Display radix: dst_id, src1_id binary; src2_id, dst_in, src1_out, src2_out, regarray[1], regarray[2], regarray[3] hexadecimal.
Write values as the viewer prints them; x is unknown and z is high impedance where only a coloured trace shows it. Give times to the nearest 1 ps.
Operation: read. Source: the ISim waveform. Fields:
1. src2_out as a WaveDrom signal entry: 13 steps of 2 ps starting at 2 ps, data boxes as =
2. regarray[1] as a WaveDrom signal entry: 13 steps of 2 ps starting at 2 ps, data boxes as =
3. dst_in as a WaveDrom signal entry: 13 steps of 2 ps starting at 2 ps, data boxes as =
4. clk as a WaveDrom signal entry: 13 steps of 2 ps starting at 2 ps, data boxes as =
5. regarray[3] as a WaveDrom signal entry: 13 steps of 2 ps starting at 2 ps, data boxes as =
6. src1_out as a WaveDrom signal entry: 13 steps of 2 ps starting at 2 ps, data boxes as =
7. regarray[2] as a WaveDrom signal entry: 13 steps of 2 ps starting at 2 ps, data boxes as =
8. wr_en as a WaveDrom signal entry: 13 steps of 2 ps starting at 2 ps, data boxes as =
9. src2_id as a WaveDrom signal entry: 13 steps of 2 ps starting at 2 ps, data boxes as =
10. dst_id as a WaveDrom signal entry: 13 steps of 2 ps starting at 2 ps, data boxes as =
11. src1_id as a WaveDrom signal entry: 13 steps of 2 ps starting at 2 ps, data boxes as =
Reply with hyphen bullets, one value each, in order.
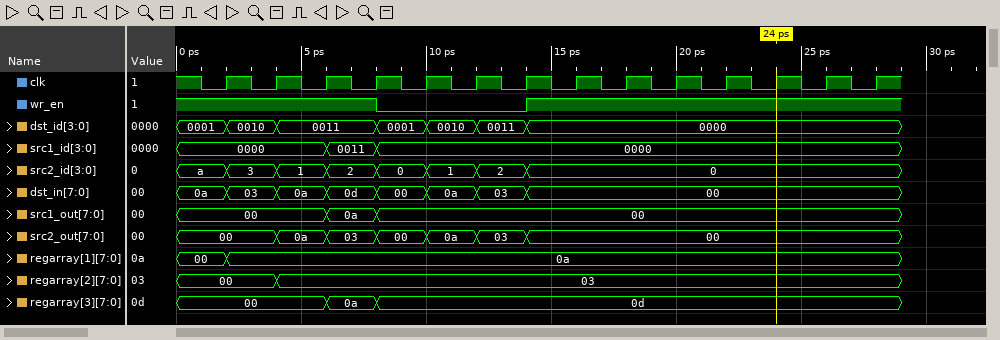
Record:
- {name: 'src2_out', wave: '=======......', data: '00 0a 03 00 0a 03 00'}
- {name: 'regarray[1]', wave: '=............', data: '0a'}
- {name: 'dst_in', wave: '=======......', data: '03 0a 0d 00 0a 03 00'}
- {name: 'clk', wave: 'p............'}
- {name: 'regarray[3]', wave: '=.==.........', data: '00 0a 0d'}
- {name: 'src1_out', wave: '=.==.........', data: '00 0a 00'}
- {name: 'regarray[2]', wave: '==...........', data: '00 03'}
- {name: 'wr_en', wave: '1..0..1......'}
- {name: 'src2_id', wave: '=======......', data: '3 1 2 0 1 2 0'}
- {name: 'dst_id', wave: '==.====......', data: '0010 0011 0001 0010 0011 0000'}
- {name: 'src1_id', wave: '=.==.........', data: '0000 0011 0000'}
